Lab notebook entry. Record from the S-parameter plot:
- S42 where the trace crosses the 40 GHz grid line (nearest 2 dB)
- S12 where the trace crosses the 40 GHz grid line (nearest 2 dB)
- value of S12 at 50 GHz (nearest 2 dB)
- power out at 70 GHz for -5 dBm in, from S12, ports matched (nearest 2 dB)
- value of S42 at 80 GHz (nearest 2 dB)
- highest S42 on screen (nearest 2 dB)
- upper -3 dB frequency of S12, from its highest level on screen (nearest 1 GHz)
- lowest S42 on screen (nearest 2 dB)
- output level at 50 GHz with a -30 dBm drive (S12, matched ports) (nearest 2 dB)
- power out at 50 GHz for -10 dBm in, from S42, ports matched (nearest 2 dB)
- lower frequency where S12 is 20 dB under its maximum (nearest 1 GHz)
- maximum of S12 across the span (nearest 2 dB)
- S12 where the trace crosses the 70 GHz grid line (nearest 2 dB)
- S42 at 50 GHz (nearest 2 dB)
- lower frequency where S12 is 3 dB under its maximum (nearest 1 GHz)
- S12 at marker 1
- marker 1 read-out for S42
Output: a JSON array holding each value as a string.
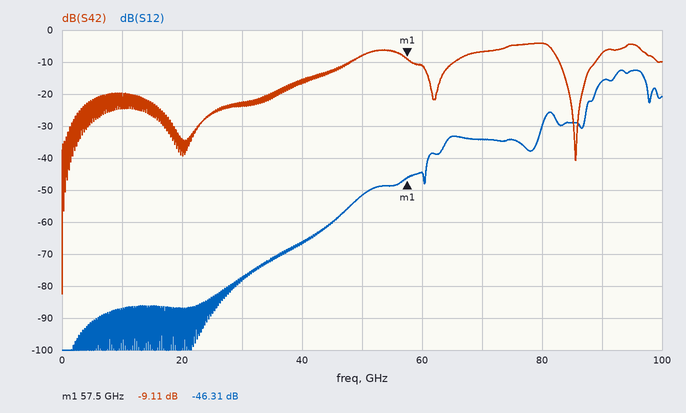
["-16 dB", "-66 dB", "-52 dB", "-40 dBm", "-4 dB", "-4 dB", "97 GHz", "-82 dB", "-82 dBm", "-18 dBm", "80 GHz", "-12 dB", "-34 dB", "-8 dB", "92 GHz", "-46.31 dB", "-9.11 dB"]
